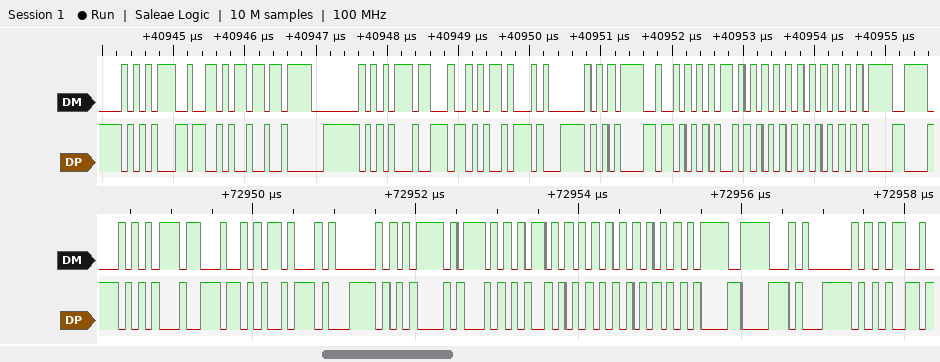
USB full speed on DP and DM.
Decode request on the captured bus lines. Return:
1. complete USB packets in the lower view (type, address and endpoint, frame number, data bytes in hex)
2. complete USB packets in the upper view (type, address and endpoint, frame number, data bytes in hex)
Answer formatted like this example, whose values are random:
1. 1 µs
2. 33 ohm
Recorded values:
1. IN ADDR 2 EP 1, DATA0 [ 00 01 00 00 ]
2. SOF 1168, IN ADDR 2 EP 1
